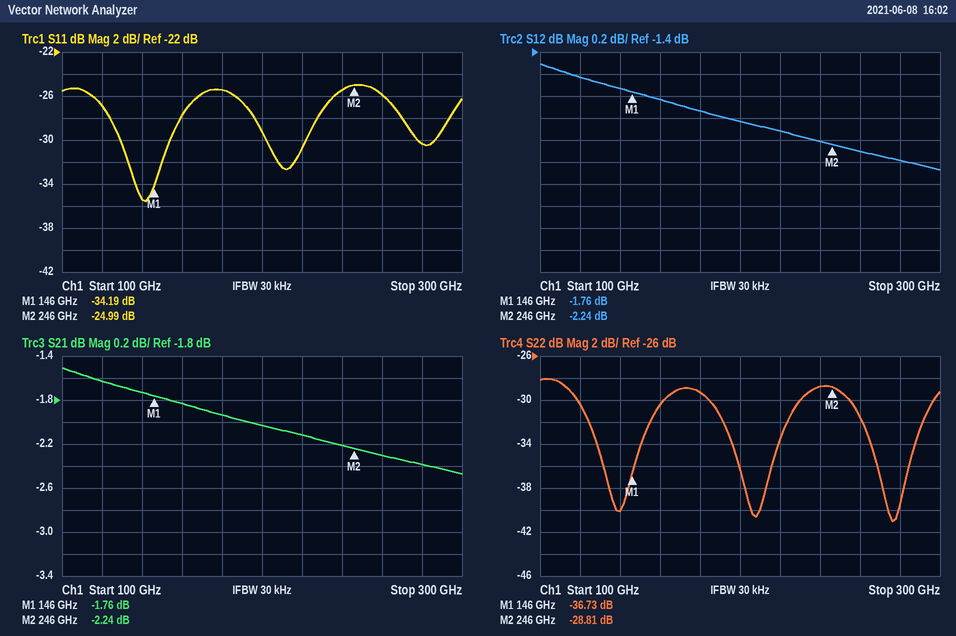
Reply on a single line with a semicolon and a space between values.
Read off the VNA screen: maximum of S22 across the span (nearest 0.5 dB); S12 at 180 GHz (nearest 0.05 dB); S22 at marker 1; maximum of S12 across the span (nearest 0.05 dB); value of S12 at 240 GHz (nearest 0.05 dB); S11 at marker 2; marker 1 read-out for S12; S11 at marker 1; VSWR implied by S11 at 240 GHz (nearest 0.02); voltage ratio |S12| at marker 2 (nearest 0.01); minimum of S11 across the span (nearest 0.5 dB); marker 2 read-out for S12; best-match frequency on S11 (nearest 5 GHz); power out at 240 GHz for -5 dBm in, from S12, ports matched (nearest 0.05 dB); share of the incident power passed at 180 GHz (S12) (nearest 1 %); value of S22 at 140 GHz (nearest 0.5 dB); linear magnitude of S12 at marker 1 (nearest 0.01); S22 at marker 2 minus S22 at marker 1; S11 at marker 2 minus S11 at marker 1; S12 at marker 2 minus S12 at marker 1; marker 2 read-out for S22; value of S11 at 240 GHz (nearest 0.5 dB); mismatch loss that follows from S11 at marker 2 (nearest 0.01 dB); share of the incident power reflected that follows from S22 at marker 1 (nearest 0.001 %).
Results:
-28.0 dB; -1.95 dB; -36.73 dB; -1.50 dB; -2.20 dB; -24.99 dB; -1.76 dB; -34.19 dB; 1.12; 0.77; -35.5 dB; -2.24 dB; 140 GHz; -7.20 dBm; 64 %; -40.0 dB; 0.82; 7.92 dB; 9.20 dB; -0.48 dB; -28.81 dB; -25.5 dB; 0.01 dB; 0.021 %
